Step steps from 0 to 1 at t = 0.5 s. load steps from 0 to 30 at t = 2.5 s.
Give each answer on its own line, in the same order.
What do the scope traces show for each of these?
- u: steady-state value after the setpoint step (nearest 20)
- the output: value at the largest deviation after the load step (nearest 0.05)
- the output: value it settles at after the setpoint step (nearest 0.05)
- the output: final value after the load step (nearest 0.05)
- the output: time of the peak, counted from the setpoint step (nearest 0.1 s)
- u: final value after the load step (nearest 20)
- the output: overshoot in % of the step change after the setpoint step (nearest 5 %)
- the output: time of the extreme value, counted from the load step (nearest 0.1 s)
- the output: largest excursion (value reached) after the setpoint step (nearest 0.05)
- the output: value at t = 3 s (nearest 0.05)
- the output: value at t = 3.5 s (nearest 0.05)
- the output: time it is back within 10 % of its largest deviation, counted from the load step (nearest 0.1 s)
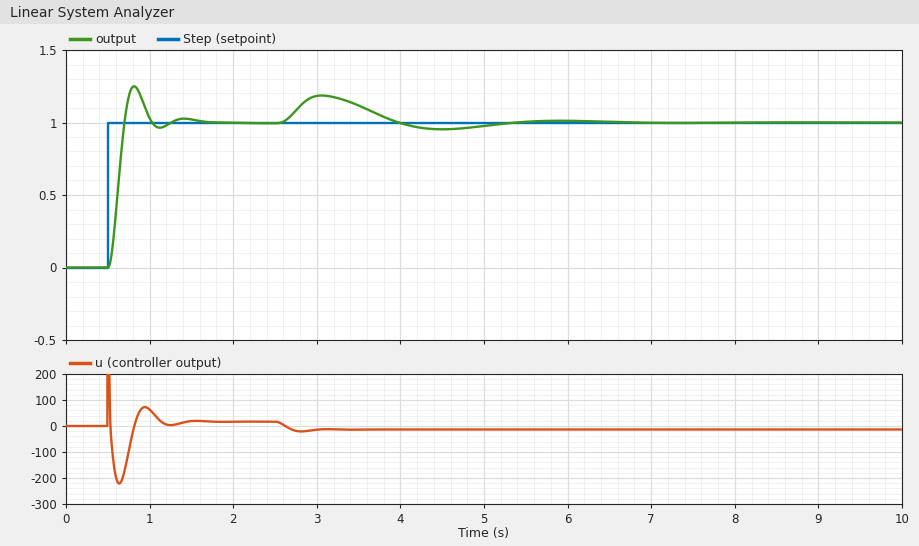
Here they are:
20
1.20
1.00
1.00
0.3 s
-20
25 %
0.6 s
1.25
1.20
1.10
2.6 s
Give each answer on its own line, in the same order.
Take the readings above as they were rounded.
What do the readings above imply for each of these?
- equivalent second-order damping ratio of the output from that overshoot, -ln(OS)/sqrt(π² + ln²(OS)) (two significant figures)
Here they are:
0.40
